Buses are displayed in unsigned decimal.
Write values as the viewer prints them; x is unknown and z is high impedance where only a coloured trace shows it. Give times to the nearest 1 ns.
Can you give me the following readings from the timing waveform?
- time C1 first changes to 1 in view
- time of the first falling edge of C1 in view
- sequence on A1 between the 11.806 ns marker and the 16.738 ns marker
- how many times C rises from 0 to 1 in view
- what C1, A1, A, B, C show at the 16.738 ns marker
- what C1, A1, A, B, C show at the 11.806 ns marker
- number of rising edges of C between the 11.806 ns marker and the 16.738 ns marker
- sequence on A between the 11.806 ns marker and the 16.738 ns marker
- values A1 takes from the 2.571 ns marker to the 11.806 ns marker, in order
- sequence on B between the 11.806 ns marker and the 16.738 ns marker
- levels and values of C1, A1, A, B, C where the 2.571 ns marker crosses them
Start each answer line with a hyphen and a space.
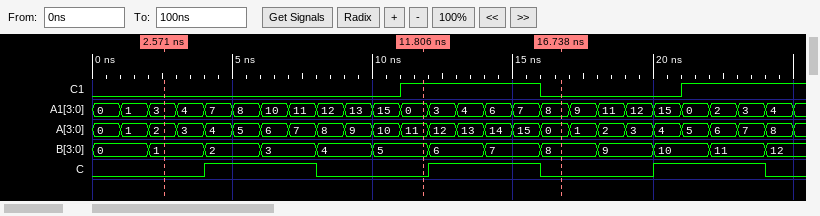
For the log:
- 11 ns
- 16 ns
- 0, 3, 4, 6, 7, 8
- 3
- C1=0, A1=8, A=0, B=8, C=0
- C1=1, A1=0, A=11, B=5, C=0
- 1
- 11, 12, 13, 14, 15, 0
- 3, 4, 7, 8, 10, 11, 12, 13, 15, 0
- 5, 6, 7, 8
- C1=0, A1=3, A=2, B=1, C=0
